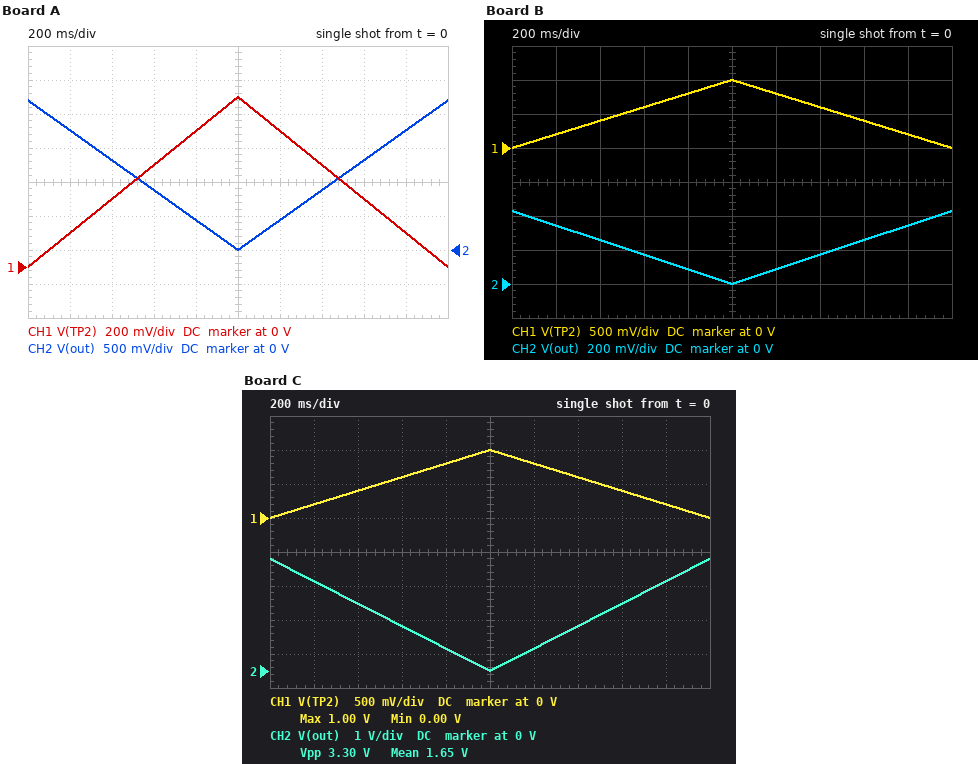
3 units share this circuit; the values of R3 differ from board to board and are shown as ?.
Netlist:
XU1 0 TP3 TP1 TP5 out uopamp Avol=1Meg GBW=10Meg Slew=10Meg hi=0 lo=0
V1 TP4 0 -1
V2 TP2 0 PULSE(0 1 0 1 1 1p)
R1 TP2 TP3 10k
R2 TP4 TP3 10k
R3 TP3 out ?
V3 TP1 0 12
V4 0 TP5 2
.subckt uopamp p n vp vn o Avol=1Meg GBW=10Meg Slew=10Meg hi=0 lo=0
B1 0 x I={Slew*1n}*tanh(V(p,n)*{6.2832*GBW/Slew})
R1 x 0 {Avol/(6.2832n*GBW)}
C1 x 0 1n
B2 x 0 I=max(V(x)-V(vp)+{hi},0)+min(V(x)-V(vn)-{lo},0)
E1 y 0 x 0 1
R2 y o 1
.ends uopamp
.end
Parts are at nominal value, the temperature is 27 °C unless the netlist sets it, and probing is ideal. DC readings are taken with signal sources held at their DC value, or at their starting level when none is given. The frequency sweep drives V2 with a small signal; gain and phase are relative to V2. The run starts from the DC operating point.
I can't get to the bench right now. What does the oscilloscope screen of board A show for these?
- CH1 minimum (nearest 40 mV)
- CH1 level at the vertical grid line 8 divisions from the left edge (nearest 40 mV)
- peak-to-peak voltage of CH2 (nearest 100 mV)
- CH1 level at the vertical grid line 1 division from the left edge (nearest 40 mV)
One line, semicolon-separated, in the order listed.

0 V; 400 mV; 2.2 V; 200 mV
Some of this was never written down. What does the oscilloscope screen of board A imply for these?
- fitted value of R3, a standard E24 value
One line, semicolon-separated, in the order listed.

22 kΩ
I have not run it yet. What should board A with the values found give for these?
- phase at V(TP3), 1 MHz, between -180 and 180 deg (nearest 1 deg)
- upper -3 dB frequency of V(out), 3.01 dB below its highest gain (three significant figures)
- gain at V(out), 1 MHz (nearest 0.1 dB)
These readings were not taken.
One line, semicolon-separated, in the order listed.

62 deg; 1.85 MHz; 5.7 dB
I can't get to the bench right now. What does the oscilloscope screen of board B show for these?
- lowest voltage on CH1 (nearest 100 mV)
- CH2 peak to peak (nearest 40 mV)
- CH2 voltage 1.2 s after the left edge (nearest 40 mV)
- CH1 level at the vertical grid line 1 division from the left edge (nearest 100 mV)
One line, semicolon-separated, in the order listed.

0 V; 440 mV; 80 mV; 200 mV
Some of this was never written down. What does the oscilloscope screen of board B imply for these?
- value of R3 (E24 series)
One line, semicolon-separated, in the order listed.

4.3 kΩ
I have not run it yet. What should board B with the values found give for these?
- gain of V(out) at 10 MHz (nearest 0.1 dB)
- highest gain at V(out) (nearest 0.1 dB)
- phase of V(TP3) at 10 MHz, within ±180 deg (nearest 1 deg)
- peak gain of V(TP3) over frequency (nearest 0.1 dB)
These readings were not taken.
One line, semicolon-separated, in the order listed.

-13.8 dB; -7.3 dB; 28 deg; -12.7 dB
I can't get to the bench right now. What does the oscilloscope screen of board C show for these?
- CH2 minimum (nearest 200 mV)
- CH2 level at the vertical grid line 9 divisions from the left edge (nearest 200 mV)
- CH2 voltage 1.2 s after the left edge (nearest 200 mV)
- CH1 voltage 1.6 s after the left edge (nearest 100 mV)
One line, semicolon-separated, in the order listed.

0 V; 2.6 V; 600 mV; 400 mV
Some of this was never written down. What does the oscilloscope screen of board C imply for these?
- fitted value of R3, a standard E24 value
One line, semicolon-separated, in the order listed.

33 kΩ
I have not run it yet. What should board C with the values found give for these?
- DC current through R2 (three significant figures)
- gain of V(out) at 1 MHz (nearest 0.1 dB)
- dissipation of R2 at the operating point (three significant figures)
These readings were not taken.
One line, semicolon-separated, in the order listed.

100 µA; 8.4 dB; 100 µW
